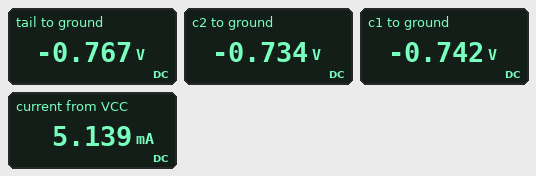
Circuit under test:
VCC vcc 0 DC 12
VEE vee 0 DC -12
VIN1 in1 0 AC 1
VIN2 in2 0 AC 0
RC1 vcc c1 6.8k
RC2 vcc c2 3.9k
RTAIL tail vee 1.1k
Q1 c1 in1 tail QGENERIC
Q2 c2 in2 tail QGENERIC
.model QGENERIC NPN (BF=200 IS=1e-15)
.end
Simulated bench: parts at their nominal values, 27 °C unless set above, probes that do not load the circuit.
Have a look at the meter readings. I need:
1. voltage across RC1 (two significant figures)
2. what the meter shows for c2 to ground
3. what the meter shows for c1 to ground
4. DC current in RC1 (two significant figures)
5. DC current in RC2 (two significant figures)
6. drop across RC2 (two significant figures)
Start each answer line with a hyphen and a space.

- 13 V
- -0.734 V
- -0.742 V
- 1.9 mA
- 3.3 mA
- 13 V
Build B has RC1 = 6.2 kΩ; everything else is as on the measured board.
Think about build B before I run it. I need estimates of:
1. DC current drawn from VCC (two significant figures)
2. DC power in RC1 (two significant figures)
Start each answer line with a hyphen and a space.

- 5.3 mA
- 26 mW
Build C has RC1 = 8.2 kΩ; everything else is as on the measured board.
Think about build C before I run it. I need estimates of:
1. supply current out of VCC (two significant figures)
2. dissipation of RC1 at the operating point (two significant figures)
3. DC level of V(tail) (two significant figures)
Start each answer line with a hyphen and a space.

- 4.8 mA
- 20 mW
- -770 mV
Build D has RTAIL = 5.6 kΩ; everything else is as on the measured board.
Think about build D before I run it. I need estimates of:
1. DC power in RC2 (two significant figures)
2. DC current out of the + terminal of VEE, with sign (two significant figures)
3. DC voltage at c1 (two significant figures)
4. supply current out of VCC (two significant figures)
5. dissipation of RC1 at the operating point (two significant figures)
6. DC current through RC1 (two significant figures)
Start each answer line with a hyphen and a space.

- 3.9 mW
- -2.0 mA
- 5.2 V
- 2.0 mA
- 6.8 mW
- 1.0 mA
